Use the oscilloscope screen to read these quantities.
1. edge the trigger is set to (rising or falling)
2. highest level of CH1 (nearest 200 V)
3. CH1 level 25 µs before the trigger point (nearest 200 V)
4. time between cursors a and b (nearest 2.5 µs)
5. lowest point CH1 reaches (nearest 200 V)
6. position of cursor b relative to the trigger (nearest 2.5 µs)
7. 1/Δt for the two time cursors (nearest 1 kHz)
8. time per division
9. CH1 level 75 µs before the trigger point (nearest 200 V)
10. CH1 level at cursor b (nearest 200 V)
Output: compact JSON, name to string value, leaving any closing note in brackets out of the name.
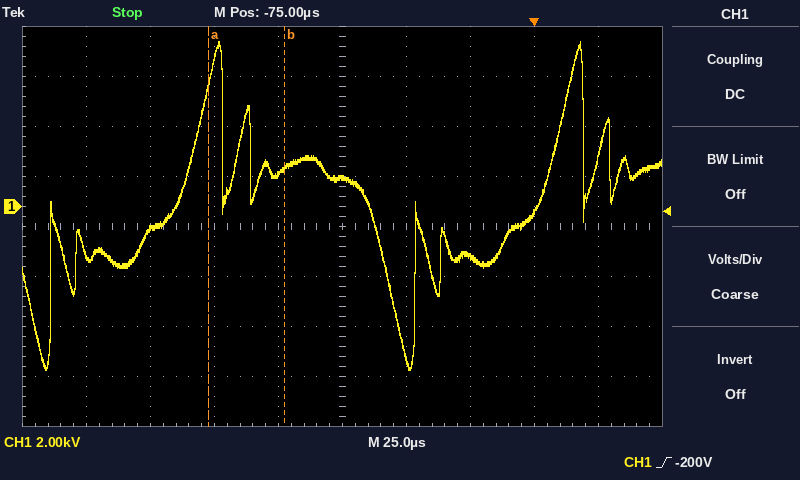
{"edge the trigger is set to": "rising", "highest level of CH1": "6.6 kV", "CH1 level 25 µs before the trigger point": "-2.0 kV", "time between cursors a and b": "30.0 µs", "lowest point CH1 reaches": "-6.6 kV", "position of cursor b relative to the trigger": "-97.5 µs", "1/Δt for the two time cursors": "33 kHz", "time per division": "25 µs", "CH1 level 75 µs before the trigger point": "1.2 kV", "CH1 level at cursor b": "1.6 kV"}
